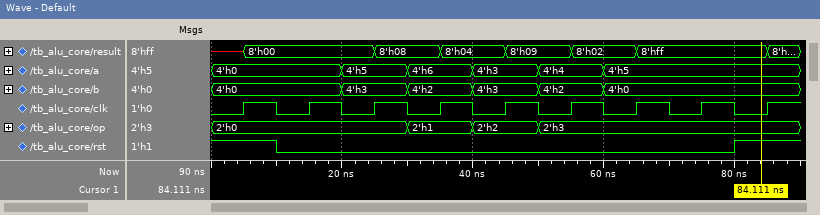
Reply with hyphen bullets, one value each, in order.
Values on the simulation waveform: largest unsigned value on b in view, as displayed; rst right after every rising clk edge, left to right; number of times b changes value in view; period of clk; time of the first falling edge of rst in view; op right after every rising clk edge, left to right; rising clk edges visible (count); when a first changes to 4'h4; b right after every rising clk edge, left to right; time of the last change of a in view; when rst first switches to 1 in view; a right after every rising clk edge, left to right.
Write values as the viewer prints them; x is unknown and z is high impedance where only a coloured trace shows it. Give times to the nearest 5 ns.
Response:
- 4'h3
- 1 0 0 0 0 0 0 0 1
- 5
- 10 ns
- 10 ns
- 2'h0, 2'h0, 2'h0, 2'h1, 2'h2, 2'h3, 2'h3, 2'h3, 2'h3
- 9
- 50 ns
- 4'h0, 4'h0, 4'h3, 4'h2, 4'h3, 4'h2, 4'h0, 4'h0, 4'h0
- 60 ns
- 80 ns
- 4'h0, 4'h0, 4'h5, 4'h6, 4'h3, 4'h4, 4'h5, 4'h5, 4'h5
